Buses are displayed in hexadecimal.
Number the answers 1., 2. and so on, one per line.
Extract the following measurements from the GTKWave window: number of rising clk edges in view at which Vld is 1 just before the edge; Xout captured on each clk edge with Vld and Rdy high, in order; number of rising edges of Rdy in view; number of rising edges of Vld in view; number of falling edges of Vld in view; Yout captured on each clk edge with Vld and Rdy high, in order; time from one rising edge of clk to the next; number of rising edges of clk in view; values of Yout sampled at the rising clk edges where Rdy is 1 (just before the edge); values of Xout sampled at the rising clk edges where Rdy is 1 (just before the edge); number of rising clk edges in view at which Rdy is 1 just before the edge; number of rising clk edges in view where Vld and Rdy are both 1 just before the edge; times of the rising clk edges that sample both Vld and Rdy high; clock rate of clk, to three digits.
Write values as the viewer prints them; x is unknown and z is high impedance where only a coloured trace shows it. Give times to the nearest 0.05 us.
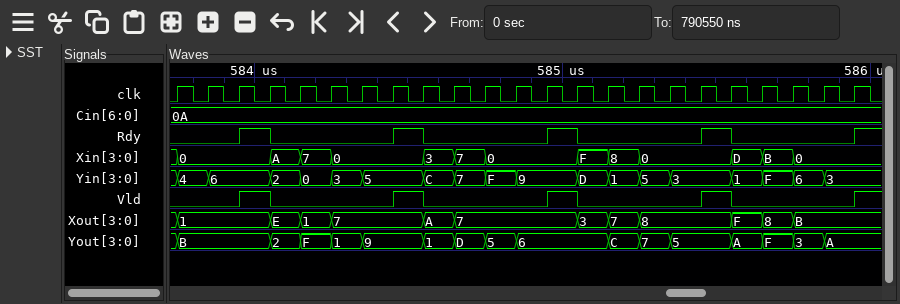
1. 4
2. 1, 7, 7, 8
3. 5
4. 5
5. 4
6. B, 9, 6, 5
7. 0.1 us
8. 23
9. B, 9, 6, 5
10. 1, 7, 7, 8
11. 4
12. 4
13. 584.05 us, 584.55 us, 585.05 us, 585.55 us
14. 10.0 MHz
